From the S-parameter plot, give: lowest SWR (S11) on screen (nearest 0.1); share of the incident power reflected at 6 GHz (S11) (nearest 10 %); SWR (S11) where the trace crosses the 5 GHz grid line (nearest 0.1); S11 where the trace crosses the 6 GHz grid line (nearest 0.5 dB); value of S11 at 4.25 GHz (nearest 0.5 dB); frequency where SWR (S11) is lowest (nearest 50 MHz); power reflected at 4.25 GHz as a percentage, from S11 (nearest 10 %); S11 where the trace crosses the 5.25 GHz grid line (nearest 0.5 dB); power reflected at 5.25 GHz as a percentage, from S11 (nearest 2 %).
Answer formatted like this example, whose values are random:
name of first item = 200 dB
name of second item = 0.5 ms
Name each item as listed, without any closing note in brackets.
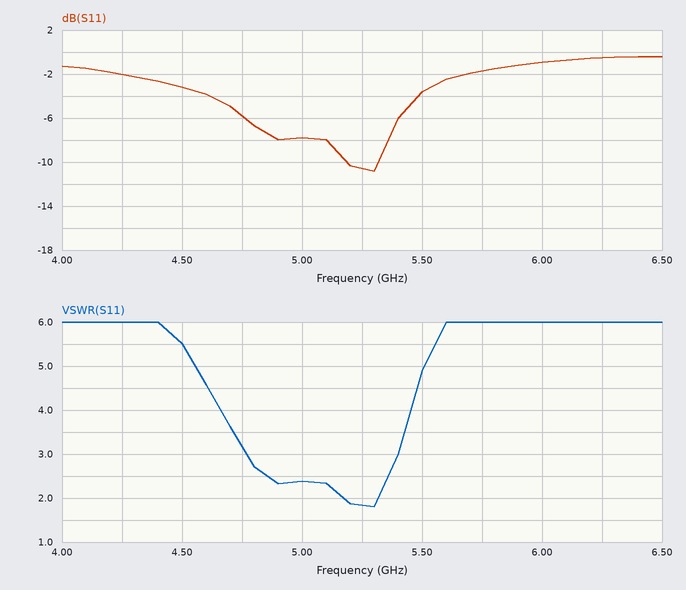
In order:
lowest SWR (S11) on screen = 1.8
share of the incident power reflected at 6 GHz (S11) = 80 %
SWR (S11) where the trace crosses the 5 GHz grid line = 2.4
S11 where the trace crosses the 6 GHz grid line = -1.0 dB
value of S11 at 4.25 GHz = -2.0 dB
frequency where SWR (S11) is lowest = 5.30 GHz
power reflected at 4.25 GHz as a percentage, from S11 = 60 %
S11 where the trace crosses the 5.25 GHz grid line = -10.5 dB
power reflected at 5.25 GHz as a percentage, from S11 = 8 %
